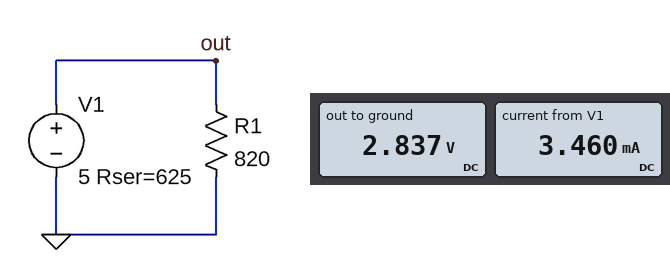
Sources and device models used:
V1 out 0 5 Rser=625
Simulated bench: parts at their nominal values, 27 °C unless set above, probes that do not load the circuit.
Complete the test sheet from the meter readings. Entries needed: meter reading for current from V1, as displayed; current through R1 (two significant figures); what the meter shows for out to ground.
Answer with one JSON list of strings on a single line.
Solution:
["3.460 mA", "3.5 mA", "2.837 V"]
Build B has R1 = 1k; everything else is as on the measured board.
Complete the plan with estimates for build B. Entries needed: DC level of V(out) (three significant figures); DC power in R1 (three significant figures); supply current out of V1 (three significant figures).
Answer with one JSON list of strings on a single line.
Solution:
["3.08 V", "9.47 mW", "3.08 mA"]
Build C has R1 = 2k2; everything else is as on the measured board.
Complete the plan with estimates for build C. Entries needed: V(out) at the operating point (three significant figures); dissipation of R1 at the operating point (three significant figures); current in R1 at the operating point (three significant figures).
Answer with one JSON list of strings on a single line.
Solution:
["3.89 V", "6.89 mW", "1.77 mA"]
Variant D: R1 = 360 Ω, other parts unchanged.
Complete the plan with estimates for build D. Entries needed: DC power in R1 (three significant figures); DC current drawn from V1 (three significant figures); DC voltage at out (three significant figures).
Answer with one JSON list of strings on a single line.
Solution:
["9.28 mW", "5.08 mA", "1.83 V"]
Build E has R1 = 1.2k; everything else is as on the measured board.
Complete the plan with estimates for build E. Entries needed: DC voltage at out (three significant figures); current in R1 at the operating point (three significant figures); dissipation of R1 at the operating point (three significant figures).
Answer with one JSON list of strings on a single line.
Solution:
["3.29 V", "2.74 mA", "9.01 mW"]
